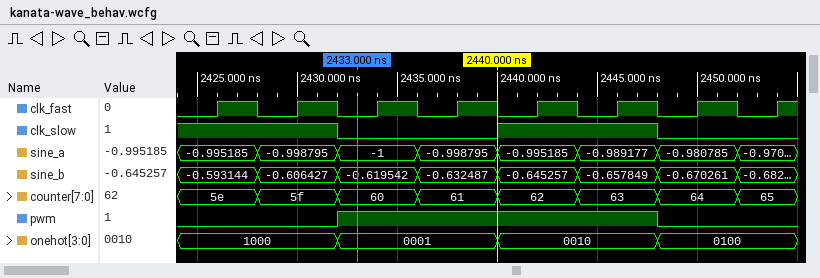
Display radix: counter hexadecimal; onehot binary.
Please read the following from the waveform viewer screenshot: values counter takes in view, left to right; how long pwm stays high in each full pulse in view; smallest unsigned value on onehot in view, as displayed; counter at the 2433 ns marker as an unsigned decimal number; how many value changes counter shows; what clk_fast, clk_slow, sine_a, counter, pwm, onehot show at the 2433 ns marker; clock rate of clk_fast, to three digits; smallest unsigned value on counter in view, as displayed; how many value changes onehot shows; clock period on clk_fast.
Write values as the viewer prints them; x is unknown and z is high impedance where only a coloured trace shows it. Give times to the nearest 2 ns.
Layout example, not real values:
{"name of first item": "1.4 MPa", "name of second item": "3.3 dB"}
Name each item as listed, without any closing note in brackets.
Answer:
{"values counter takes in view, left to right": "5e, 5f, 60, 61, 62, 63, 64, 65", "how long pwm stays high in each full pulse in view": "16 ns", "smallest unsigned value on onehot in view, as displayed": "0001", "counter at the 2433 ns marker as an unsigned decimal number": "96", "how many value changes counter shows": "7", "what clk_fast, clk_slow, sine_a, counter, pwm, onehot show at the 2433 ns marker": "clk_fast=0, clk_slow=0, sine_a=-1, counter=60, pwm=1, onehot=0001", "clock rate of clk_fast, to three digits": "250 MHz", "smallest unsigned value on counter in view, as displayed": "5e", "how many value changes onehot shows": "3", "clock period on clk_fast": "4 ns"}
